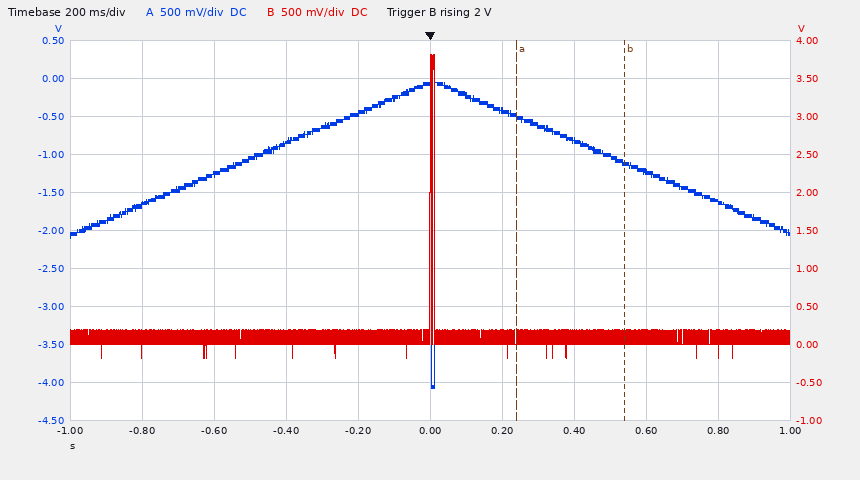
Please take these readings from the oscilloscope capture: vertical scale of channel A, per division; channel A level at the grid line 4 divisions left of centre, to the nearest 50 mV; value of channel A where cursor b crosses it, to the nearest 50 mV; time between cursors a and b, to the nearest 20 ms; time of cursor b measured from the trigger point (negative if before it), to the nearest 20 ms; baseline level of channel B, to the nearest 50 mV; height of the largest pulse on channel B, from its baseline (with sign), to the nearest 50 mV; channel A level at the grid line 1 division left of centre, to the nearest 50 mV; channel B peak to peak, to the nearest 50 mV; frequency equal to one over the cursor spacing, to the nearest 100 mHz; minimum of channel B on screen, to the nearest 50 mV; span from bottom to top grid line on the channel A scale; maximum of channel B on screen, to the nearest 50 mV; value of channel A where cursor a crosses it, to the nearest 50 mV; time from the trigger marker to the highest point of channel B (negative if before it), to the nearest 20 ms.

500 mV
-1.65 V
-1.10 V
300 ms
+540 ms
100 mV
+3.70 V
-450 mV
4.00 V
3.3 Hz
-200 mV
5 V
3.80 V
-500 mV
0 ms
